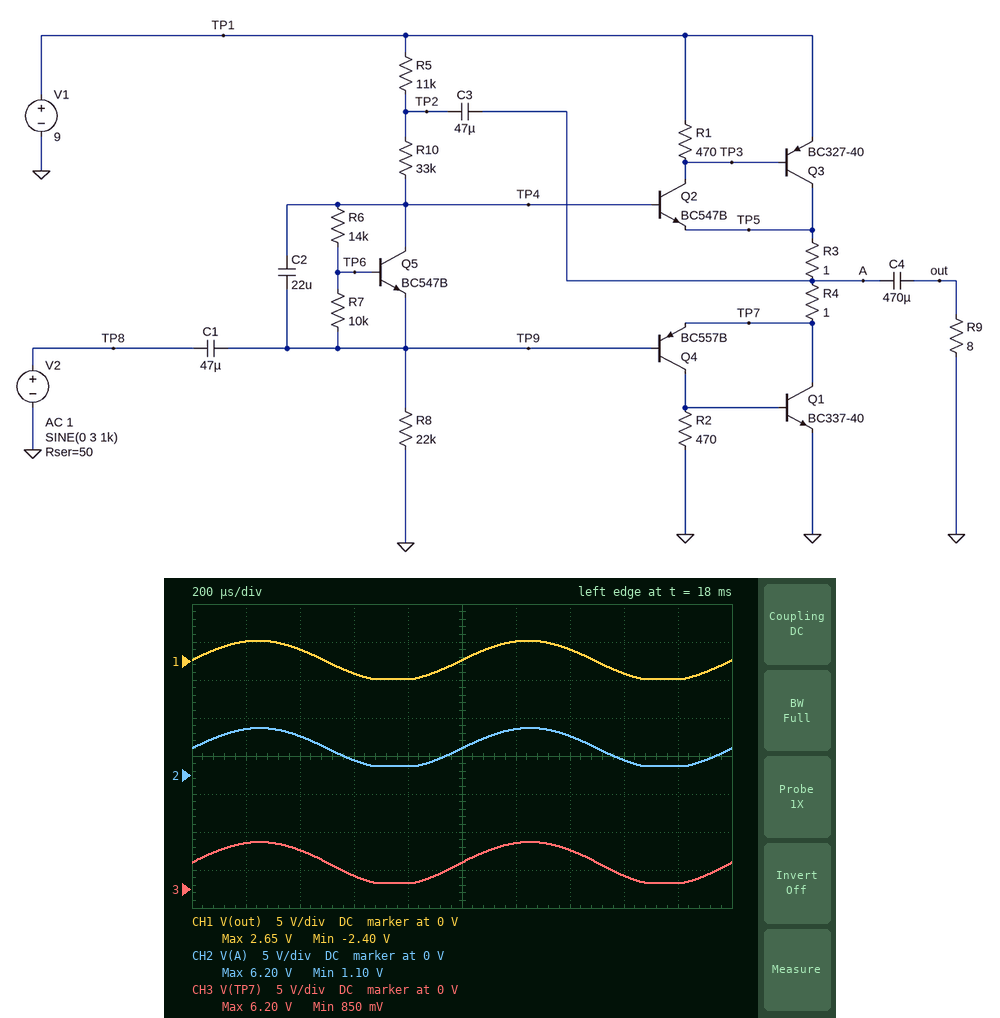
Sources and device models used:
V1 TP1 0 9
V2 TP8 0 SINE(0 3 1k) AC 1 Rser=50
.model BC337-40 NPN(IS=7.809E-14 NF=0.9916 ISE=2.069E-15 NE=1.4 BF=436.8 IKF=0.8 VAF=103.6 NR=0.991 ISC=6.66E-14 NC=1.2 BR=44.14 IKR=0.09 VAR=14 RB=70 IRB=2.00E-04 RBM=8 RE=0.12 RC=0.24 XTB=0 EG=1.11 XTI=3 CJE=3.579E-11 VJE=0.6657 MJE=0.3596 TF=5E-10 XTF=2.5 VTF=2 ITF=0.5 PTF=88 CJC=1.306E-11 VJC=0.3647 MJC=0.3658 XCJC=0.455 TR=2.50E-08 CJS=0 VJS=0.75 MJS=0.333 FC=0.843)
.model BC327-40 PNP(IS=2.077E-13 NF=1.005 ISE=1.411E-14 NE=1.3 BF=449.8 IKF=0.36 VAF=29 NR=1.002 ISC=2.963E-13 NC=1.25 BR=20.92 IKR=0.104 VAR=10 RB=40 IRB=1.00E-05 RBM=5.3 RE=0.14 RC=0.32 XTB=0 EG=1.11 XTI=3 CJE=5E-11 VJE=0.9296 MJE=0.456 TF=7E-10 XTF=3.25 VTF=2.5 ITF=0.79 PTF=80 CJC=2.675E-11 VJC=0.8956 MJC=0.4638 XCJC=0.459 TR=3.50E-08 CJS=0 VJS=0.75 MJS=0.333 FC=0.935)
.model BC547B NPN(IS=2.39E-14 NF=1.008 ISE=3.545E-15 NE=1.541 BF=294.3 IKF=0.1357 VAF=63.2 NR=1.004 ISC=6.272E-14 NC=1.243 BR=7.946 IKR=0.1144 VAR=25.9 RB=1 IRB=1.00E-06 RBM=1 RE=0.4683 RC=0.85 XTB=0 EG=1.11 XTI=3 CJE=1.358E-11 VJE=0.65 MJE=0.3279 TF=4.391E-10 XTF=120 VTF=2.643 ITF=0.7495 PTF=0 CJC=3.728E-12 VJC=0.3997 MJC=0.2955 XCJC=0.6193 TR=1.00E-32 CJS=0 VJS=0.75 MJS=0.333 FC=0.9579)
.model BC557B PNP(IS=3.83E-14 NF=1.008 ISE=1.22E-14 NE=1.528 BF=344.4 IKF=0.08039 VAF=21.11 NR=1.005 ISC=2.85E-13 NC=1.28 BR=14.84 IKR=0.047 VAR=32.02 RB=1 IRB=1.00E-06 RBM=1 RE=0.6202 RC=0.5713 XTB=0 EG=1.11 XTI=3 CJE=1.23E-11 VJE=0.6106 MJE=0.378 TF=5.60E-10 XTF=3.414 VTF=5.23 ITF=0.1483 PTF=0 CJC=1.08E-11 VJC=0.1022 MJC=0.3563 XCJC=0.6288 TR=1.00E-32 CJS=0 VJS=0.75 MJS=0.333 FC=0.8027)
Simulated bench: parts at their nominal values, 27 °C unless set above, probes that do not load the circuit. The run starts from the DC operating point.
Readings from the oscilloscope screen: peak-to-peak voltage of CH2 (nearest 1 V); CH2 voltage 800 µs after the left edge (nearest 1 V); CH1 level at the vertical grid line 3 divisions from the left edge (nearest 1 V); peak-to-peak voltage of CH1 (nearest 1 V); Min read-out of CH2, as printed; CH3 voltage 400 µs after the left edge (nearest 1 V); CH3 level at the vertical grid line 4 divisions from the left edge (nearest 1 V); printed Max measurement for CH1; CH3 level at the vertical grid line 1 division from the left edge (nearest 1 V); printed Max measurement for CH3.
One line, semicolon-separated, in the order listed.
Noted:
5 V; 1 V; -2 V; 5 V; 1.10 V; 5 V; 1 V; 2.65 V; 6 V; 6.20 V
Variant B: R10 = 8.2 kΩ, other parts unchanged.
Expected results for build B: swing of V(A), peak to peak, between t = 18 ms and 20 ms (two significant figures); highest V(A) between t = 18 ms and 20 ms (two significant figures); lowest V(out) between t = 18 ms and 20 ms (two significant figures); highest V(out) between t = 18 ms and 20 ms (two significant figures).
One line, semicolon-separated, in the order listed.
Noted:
5.4 V; 7.4 V; -2.7 V; 2.7 V
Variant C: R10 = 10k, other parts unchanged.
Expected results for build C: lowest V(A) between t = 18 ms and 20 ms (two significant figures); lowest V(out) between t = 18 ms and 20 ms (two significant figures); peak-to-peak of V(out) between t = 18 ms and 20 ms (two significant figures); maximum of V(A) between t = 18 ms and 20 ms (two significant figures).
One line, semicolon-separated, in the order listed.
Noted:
1.9 V; -2.7 V; 5.4 V; 7.3 V
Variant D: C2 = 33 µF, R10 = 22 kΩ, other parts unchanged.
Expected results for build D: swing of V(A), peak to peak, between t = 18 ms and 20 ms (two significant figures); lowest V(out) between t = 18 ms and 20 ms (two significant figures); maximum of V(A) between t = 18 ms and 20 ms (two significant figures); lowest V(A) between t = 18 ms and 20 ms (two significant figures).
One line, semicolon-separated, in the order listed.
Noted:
5.3 V; -2.6 V; 6.4 V; 1.2 V
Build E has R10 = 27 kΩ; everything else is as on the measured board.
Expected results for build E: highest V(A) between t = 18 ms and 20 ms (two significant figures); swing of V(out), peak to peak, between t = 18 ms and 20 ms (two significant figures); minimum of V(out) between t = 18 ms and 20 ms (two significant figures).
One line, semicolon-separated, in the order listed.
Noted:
6.3 V; 5.2 V; -2.5 V
